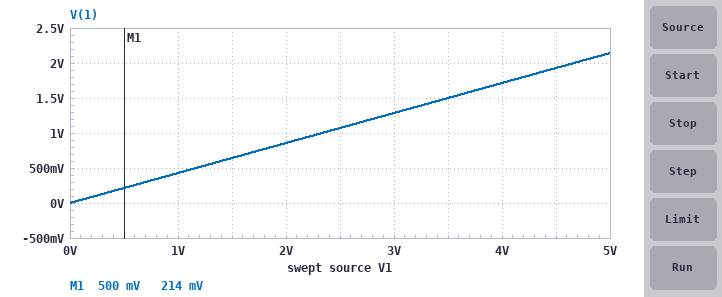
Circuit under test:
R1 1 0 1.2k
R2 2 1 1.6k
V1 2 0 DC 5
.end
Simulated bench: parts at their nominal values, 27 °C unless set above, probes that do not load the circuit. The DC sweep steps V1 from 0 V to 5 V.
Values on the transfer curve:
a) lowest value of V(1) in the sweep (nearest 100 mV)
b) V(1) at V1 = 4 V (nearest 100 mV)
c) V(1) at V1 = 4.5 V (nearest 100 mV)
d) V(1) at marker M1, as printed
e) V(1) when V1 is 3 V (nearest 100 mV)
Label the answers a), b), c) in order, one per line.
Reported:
a) 0 V
b) 1.7 V
c) 1.9 V
d) 214 mV
e) 1.3 V
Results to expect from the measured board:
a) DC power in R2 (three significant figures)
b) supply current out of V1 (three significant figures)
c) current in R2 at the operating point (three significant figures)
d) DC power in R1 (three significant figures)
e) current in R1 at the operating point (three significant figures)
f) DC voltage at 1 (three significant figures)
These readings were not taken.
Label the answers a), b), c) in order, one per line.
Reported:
a) 5.10 mW
b) 1.79 mA
c) 1.79 mA
d) 3.83 mW
e) 1.79 mA
f) 2.14 V
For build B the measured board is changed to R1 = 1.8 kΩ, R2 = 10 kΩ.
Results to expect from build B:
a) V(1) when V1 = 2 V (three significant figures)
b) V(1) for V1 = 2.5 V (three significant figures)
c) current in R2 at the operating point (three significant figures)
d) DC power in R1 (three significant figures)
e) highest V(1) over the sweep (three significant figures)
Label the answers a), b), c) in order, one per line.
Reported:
a) 305 mV
b) 381 mV
c) 424 µA
d) 323 µW
e) 763 mV
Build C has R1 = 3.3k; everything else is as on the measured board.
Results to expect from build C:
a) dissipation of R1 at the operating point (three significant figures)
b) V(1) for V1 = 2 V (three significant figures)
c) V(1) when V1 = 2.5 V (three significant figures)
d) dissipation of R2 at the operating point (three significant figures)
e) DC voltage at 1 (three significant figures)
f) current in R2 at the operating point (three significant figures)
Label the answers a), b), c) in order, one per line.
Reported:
a) 3.44 mW
b) 1.35 V
c) 1.68 V
d) 1.67 mW
e) 3.37 V
f) 1.02 mA
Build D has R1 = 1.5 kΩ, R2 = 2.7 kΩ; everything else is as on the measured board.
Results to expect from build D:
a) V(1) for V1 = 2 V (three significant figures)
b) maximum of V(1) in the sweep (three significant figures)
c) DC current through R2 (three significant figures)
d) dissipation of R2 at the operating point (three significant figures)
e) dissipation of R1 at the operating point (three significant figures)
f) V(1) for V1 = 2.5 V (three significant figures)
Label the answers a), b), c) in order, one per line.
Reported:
a) 714 mV
b) 1.79 V
c) 1.19 mA
d) 3.83 mW
e) 2.13 mW
f) 893 mV
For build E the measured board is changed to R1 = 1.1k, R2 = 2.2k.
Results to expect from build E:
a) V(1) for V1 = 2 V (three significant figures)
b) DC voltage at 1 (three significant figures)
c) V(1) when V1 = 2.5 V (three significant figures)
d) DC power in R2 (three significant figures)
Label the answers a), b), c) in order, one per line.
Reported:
a) 667 mV
b) 1.67 V
c) 833 mV
d) 5.05 mW
